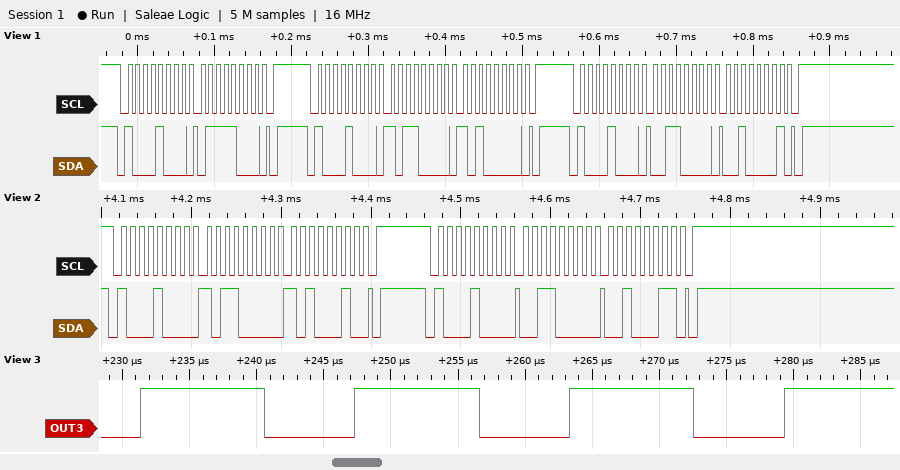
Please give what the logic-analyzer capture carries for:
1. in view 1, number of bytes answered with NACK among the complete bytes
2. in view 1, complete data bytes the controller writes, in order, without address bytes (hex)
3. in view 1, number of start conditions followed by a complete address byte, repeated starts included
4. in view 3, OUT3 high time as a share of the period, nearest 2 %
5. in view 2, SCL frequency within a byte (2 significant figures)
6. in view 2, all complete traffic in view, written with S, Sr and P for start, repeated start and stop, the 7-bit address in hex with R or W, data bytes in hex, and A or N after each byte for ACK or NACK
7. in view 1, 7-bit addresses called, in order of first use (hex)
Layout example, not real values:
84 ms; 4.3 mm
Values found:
0; 78 B0 A0 30 21; 3; 58 %; 100 kHz; S 44W A B0 A A2 A P S 44W A 30 A 23 A P; 0x44
